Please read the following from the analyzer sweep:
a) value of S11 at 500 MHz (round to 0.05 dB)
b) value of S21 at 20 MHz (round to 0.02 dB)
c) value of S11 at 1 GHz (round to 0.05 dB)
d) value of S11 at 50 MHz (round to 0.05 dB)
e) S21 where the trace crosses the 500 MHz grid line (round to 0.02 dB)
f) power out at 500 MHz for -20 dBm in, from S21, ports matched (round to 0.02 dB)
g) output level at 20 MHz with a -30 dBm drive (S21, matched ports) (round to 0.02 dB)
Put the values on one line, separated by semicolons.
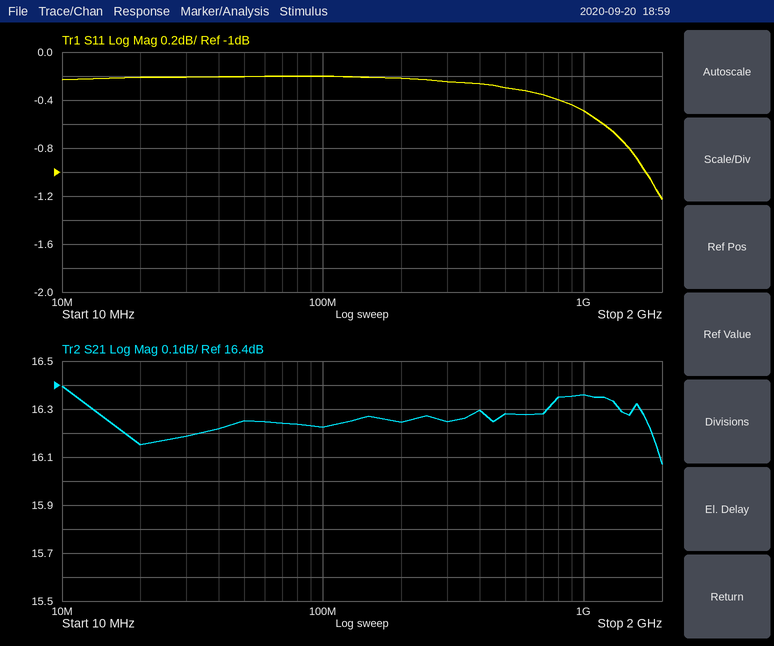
-0.30 dB; 16.16 dB; -0.50 dB; -0.20 dB; 16.28 dB; -3.72 dBm; -13.84 dBm
